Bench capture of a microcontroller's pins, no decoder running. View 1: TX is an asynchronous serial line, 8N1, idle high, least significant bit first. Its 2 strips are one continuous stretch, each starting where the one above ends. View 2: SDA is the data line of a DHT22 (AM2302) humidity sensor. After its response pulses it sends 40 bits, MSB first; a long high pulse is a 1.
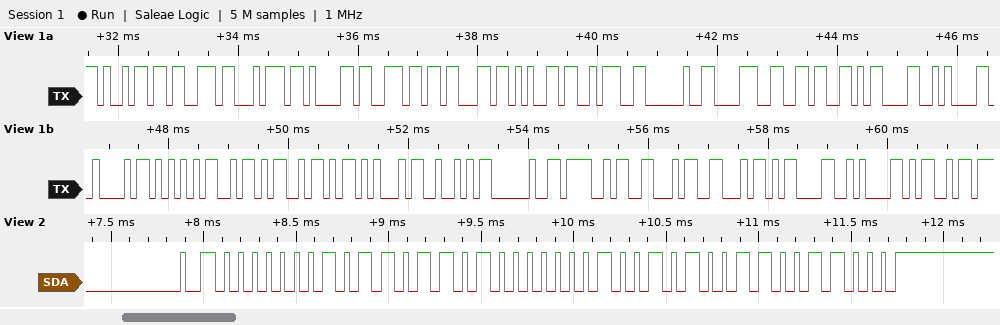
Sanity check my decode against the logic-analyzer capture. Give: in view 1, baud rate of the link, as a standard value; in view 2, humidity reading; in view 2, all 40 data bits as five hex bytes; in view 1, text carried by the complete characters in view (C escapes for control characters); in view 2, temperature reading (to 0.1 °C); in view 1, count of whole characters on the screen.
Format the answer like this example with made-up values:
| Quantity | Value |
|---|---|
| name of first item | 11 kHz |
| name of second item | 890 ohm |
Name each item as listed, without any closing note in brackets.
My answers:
| Quantity | Value |
|---|---|
| in view 1, baud rate of the link, as a standard value | 9600 baud |
| in view 2, humidity reading | 36.5 % |
| in view 2, all 40 data bits as five hex bytes | 01 6D 01 29 98 |
| in view 1, text carried by the complete characters in view | "istance: 86\r\nBUZZER OFF\r\nM" |
| in view 2, temperature reading | 29.7 °C |
| in view 1, count of whole characters on the screen | 26 |
